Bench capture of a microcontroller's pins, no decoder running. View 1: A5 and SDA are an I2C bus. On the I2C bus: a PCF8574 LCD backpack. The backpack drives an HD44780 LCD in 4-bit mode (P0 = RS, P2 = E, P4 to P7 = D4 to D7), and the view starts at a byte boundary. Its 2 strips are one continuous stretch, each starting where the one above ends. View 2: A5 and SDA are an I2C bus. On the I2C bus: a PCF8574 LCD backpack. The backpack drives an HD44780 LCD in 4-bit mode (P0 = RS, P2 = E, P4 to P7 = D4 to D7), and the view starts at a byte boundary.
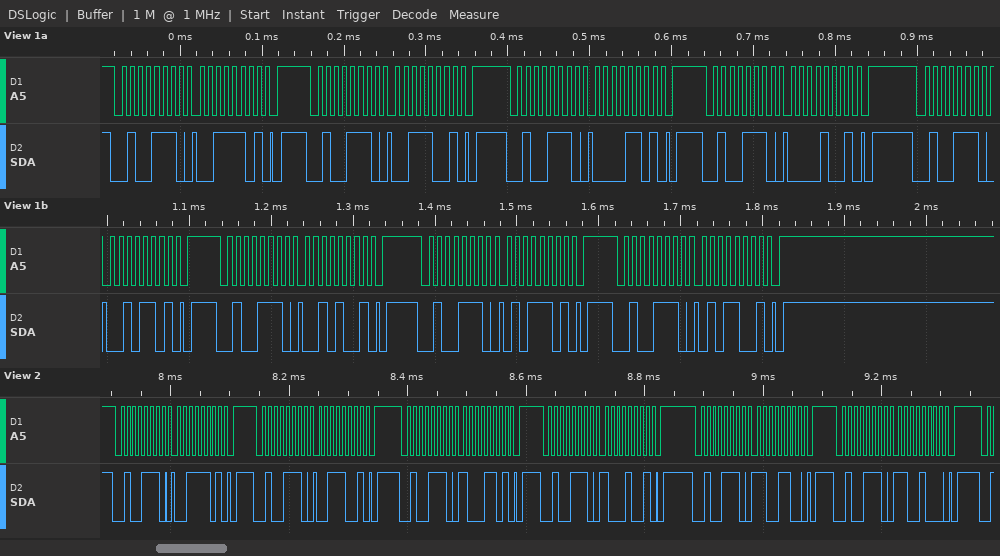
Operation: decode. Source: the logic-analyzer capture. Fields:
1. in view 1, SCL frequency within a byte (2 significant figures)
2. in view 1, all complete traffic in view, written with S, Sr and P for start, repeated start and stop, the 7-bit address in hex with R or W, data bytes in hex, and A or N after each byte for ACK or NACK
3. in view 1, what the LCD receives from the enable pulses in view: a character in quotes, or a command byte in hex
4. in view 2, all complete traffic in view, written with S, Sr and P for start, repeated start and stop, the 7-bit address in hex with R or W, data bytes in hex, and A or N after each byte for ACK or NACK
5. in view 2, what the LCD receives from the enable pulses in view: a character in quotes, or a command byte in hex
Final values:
100 kHz
S 27W A 3D A P S 27W A 39 A P S 27W A 0D A P S 27W A 09 A P S 27W A 2D A P S 27W A 29 A P S 27W A 5D A P S 27W A 59 A P
'0' '%'
S 27W A 3D A P S 27W A 39 A P S 27W A 8D A P S 27W A 89 A P S 27W A CC A P S 27W A C8 A P
'8'
